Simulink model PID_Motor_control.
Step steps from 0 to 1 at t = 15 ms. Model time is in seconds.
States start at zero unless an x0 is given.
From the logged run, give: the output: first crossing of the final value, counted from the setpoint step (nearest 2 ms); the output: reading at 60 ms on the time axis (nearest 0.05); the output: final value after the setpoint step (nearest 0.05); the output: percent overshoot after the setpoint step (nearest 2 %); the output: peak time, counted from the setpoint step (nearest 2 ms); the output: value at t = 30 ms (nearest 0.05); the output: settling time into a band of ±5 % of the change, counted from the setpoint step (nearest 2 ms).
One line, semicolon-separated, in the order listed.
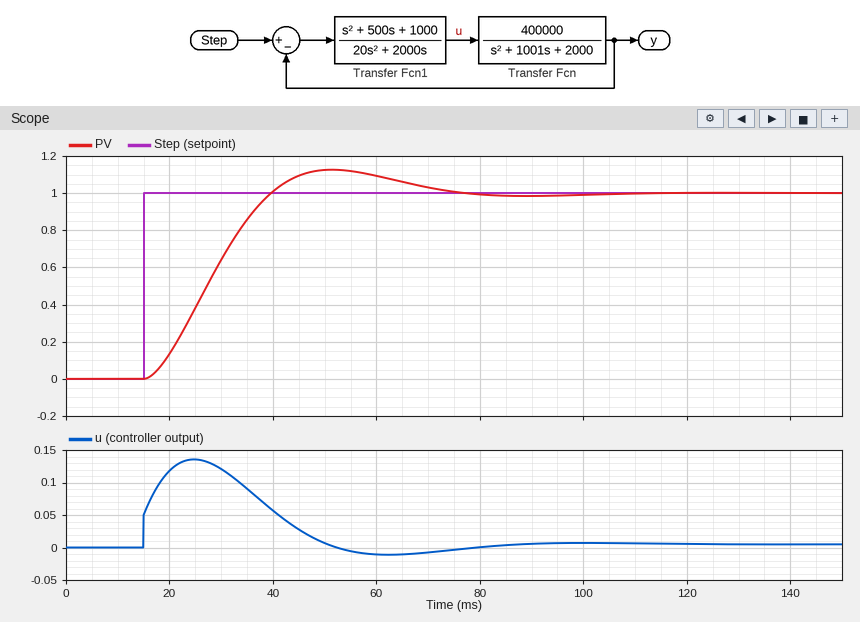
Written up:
24 ms; 1.10; 1.00; 12 %; 36 ms; 0.65; 52 ms
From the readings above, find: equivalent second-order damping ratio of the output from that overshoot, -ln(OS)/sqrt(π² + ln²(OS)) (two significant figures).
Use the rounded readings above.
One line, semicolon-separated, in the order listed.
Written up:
0.56
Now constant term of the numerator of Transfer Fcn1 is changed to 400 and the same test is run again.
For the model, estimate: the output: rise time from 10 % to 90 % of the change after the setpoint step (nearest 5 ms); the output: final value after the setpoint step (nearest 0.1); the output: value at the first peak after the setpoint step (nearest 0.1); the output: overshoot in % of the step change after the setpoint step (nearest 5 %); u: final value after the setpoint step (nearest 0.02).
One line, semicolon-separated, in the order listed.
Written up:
15 ms; 1.0; 1.1; 10 %; 0.00
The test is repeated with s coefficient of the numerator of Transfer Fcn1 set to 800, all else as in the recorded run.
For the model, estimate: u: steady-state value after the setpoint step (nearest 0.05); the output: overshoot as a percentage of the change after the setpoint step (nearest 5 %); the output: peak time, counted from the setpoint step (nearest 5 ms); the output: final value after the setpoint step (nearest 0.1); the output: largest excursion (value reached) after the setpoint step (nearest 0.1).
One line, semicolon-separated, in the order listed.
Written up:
0.00; 25 %; 25 ms; 1.0; 1.2
